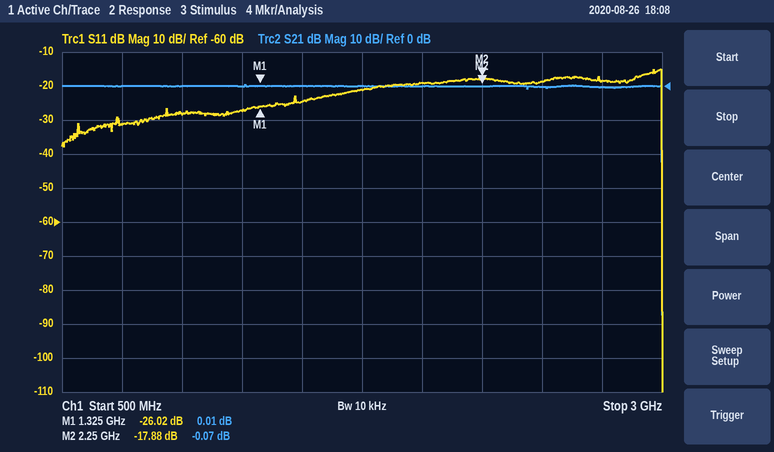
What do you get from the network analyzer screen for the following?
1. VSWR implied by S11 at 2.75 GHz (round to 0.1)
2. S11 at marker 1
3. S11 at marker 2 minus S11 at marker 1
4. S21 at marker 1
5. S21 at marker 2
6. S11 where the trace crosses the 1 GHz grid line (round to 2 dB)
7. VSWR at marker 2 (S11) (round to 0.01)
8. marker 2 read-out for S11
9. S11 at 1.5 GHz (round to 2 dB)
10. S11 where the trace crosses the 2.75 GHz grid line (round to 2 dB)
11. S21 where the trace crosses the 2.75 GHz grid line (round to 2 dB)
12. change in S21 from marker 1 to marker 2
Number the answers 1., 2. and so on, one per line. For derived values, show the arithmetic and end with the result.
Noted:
1. |Γ| = 10^(-18/20) = 0.1259; VSWR = (1 + 0.1259)/(1 − 0.1259) ≈ 1.3
2. -26.02 dB
3. -17.88 − (-26.02) = 8.14 dB
4. 0.01 dB
5. -0.07 dB
6. -28 dB
7. (1 + 0.1276)/(1 − 0.1276) ≈ 1.29
8. -17.88 dB
9. -24 dB
10. -18 dB
11. 0 dB
12. -0.07 − (0.01) = -0.08 dB
